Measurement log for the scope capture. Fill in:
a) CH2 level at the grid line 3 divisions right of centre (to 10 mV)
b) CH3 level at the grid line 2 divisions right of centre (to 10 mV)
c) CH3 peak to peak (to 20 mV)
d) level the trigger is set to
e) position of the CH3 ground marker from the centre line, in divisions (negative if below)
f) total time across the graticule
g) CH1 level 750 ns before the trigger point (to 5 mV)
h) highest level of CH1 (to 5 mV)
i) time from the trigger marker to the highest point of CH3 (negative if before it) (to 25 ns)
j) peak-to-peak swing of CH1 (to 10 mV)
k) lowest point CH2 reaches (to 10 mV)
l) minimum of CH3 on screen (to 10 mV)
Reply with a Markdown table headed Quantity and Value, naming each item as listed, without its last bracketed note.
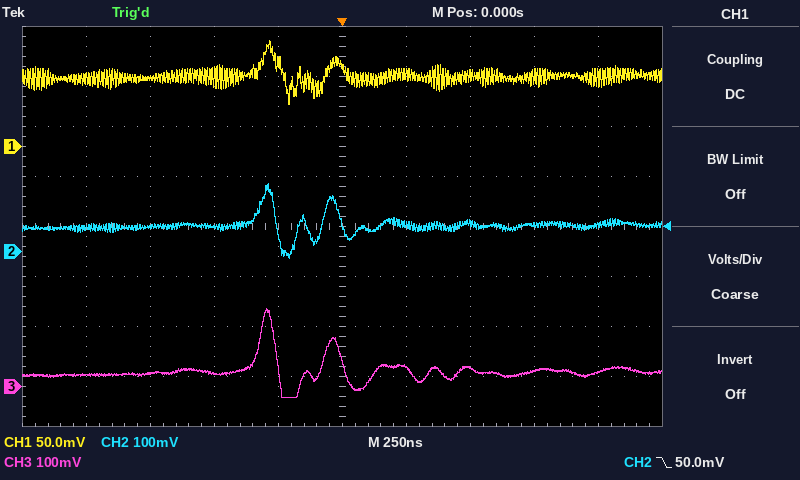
| Quantity | Value |
|---|---|
| CH2 level at the grid line 3 divisions right of centre | 50 mV |
| CH3 level at the grid line 2 divisions right of centre | 40 mV |
| CH3 peak to peak | 180 mV |
| level the trigger is set to | 50.0 mV |
| position of the CH3 ground marker from the centre line, in divisions | -3.2 div |
| total time across the graticule | 2.5 µs |
| CH1 level 750 ns before the trigger point | 70 mV |
| highest level of CH1 | 105 mV |
| time from the trigger marker to the highest point of CH3 (negative if before it) | -300 ns |
| peak-to-peak swing of CH1 | 60 mV |
| lowest point CH2 reaches | -10 mV |
| minimum of CH3 on screen | -20 mV |
